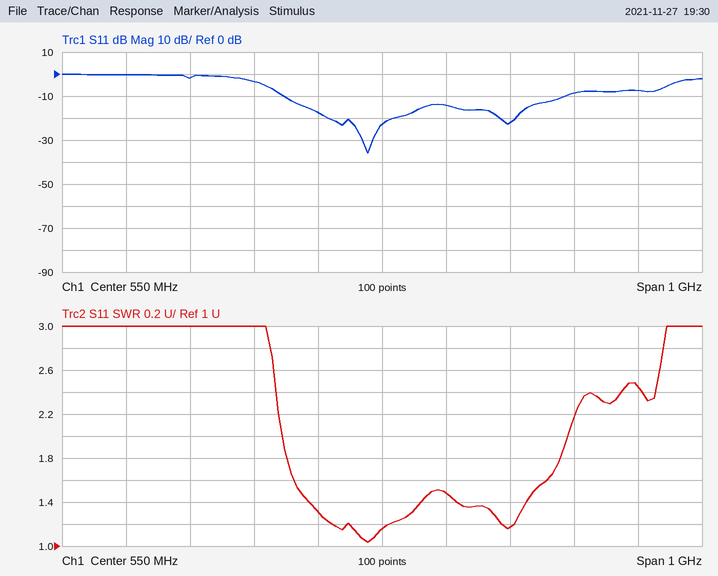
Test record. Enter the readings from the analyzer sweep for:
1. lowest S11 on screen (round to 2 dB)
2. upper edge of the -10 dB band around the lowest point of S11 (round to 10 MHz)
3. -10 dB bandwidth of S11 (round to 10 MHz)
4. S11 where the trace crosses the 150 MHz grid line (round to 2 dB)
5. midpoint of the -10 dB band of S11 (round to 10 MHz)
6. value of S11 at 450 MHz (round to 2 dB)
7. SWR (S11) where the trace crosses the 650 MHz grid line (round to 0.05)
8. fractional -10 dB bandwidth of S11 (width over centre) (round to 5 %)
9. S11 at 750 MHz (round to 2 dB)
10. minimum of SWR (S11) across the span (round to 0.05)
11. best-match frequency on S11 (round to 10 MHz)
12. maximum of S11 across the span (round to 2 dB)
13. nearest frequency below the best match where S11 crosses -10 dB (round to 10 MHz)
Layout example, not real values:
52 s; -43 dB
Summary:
-36 dB; 840 MHz; 440 MHz; 0 dB; 620 MHz; -18 dB; 1.50; 70 %; -22 dB; 1.05; 530 MHz; 0 dB; 400 MHz
